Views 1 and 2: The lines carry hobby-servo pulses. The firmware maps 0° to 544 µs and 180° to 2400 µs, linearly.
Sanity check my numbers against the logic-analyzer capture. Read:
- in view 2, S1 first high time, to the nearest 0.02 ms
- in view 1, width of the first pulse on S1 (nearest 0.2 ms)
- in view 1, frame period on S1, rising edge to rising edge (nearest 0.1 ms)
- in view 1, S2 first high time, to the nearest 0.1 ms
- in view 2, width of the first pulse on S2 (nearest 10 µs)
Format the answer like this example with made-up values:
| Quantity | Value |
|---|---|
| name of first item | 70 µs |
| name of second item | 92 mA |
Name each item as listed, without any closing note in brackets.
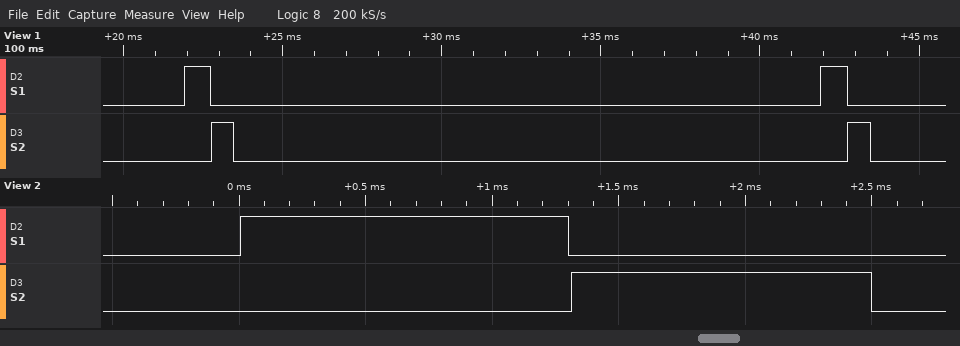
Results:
| Quantity | Value |
|---|---|
| in view 2, S1 first high time, to the nearest 0.02 ms | 1.30 ms |
| in view 1, width of the first pulse on S1 | 0.8 ms |
| in view 1, frame period on S1, rising edge to rising edge | 20.0 ms |
| in view 1, S2 first high time, to the nearest 0.1 ms | 0.7 ms |
| in view 2, width of the first pulse on S2 | 1180 µs |
